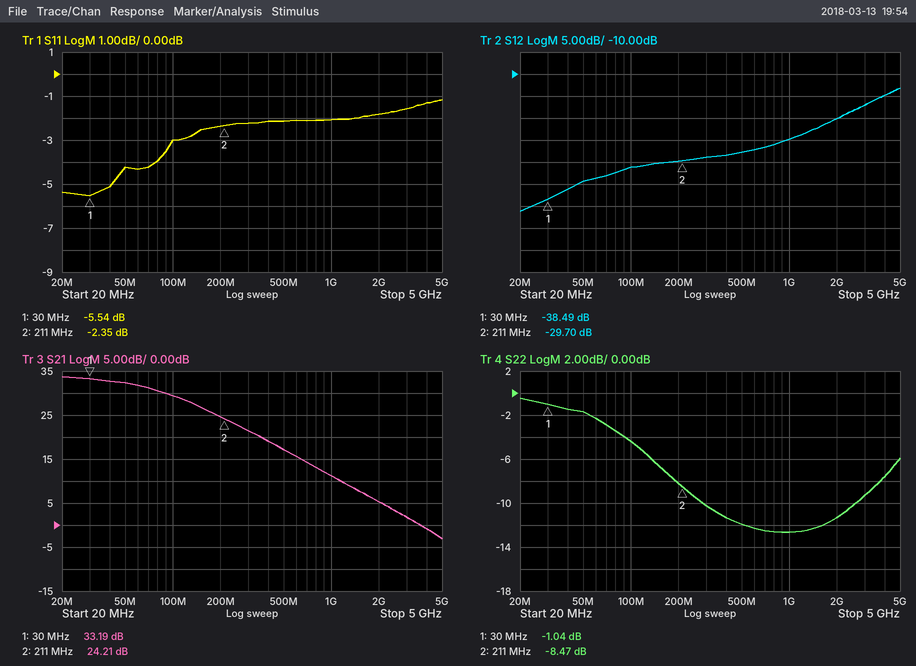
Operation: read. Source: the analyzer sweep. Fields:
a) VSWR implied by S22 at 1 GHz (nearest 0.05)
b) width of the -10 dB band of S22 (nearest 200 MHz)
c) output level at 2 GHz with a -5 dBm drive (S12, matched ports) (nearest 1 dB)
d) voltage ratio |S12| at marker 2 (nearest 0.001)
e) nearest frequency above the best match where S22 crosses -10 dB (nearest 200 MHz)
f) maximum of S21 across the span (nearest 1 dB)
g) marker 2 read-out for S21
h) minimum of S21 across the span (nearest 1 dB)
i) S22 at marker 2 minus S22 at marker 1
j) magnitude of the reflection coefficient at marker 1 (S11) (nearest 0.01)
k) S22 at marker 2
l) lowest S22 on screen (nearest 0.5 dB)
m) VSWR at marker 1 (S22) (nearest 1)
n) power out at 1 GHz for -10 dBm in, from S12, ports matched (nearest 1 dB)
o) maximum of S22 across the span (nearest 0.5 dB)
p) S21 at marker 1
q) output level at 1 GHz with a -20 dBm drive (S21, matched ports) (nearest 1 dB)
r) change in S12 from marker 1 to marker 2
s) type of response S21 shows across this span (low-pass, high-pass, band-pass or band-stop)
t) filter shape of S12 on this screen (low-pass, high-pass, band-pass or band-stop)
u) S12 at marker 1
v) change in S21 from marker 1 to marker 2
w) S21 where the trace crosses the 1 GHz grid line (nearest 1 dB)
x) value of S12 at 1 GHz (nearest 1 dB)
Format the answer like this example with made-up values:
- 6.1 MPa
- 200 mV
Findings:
- 1.60
- 2.4 GHz
- -25 dBm
- 0.033
- 2.6 GHz
- 34 dB
- 24.21 dB
- -3 dB
- -7.43 dB
- 0.53
- -8.47 dB
- -12.5 dB
- 17
- -35 dBm
- -0.5 dB
- 33.19 dB
- -9 dBm
- 8.79 dB
- low-pass
- high-pass
- -38.49 dB
- -8.98 dB
- 11 dB
- -25 dB
